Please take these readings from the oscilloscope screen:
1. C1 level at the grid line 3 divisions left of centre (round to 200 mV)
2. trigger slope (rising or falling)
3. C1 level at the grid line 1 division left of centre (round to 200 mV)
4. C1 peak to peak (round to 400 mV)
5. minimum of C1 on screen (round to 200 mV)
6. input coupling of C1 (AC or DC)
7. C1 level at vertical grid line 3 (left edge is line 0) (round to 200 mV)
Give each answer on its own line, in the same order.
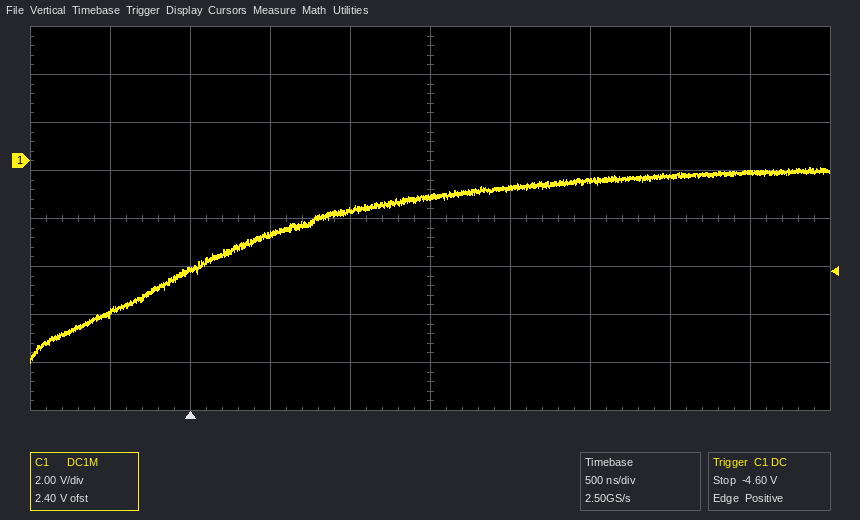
-4.6 V
rising
-2.0 V
8.0 V
-8.4 V
DC
-3.0 V
